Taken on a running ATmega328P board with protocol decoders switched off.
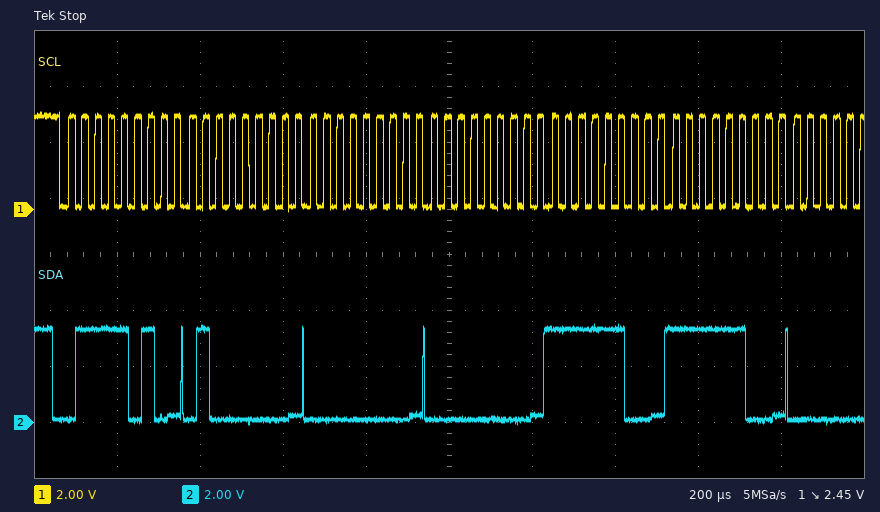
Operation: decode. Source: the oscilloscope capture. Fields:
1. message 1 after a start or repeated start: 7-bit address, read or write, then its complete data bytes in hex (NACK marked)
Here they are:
0x3D write: 40 00 00 FC FC
